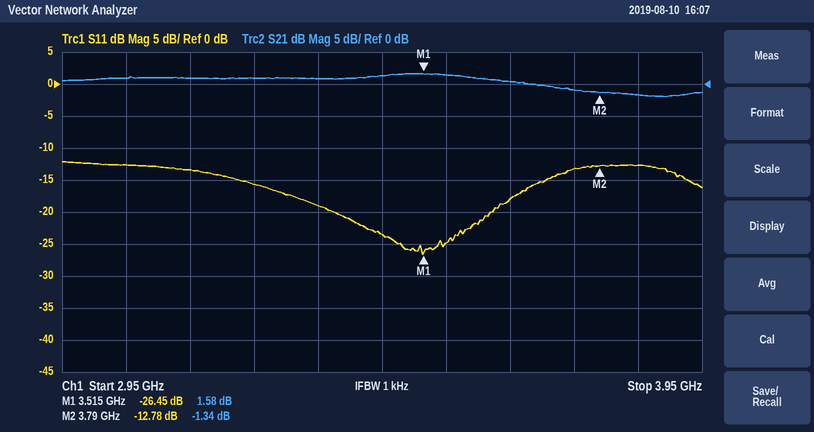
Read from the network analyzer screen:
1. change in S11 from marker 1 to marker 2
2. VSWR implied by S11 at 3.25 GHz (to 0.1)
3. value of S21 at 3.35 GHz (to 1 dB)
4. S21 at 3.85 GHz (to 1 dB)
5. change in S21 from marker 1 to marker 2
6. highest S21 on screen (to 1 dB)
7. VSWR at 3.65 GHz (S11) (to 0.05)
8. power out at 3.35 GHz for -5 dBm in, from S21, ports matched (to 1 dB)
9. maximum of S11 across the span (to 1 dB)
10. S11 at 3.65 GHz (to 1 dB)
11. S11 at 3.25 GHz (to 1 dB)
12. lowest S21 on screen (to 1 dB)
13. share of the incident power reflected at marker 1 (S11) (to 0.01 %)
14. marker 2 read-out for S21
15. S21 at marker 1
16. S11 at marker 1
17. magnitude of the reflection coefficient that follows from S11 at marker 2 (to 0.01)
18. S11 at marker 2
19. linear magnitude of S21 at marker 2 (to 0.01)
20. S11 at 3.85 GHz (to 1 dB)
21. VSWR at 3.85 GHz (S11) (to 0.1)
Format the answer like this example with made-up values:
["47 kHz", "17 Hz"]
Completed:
["13.67 dB", "1.4", "1 dB", "-2 dB", "-2.92 dB", "2 dB", "1.30", "-4 dBm", "-12 dB", "-18 dB", "-16 dB", "-2 dB", "0.23 %", "-1.34 dB", "1.58 dB", "-26.45 dB", "0.23", "-12.78 dB", "0.86", "-13 dB", "1.6"]
